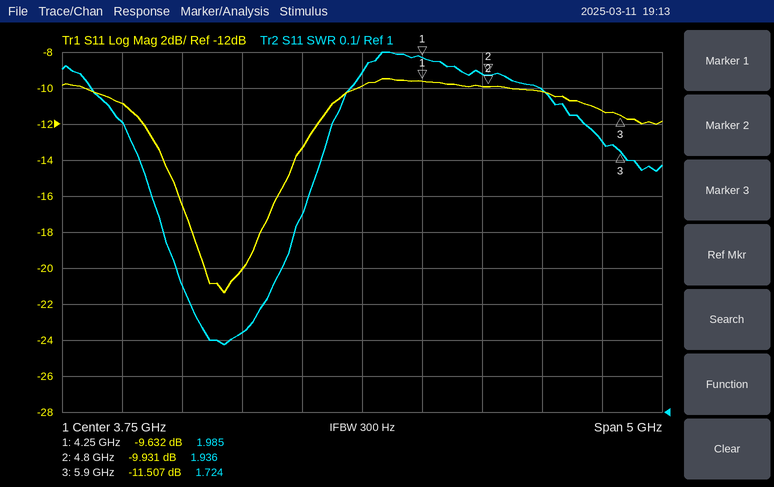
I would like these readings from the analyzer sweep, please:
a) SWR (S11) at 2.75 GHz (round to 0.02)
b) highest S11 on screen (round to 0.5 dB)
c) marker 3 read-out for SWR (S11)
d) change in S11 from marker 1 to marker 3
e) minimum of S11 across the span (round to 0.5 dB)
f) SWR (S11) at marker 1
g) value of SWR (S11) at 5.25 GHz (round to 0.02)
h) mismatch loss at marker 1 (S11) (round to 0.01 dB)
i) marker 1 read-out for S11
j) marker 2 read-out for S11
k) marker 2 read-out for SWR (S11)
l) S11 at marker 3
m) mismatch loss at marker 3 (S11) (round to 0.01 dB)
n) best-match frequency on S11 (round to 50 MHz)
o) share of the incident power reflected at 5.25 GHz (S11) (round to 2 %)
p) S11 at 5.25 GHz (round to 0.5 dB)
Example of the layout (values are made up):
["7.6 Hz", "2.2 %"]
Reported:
["1.22", "-9.5 dB", "1.724", "-1.875 dB", "-21.5 dB", "1.985", "1.90", "0.50 dB", "-9.632 dB", "-9.931 dB", "1.936", "-11.507 dB", "0.32 dB", "2.60 GHz", "10 %", "-10.0 dB"]
